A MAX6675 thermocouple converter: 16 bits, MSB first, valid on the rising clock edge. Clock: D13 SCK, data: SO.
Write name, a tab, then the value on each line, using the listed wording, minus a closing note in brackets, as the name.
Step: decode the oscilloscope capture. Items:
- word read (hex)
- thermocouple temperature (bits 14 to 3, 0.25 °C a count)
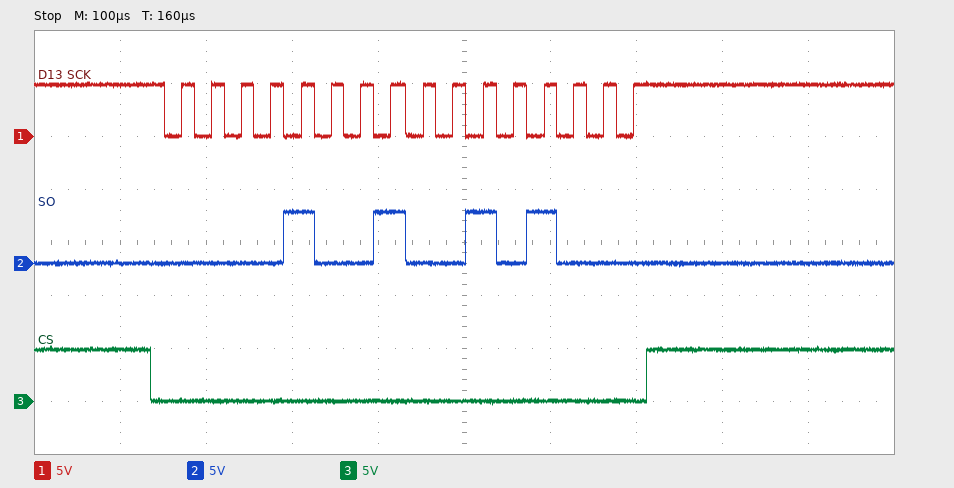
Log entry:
word read	0x0928
thermocouple temperature	73.25 °C
